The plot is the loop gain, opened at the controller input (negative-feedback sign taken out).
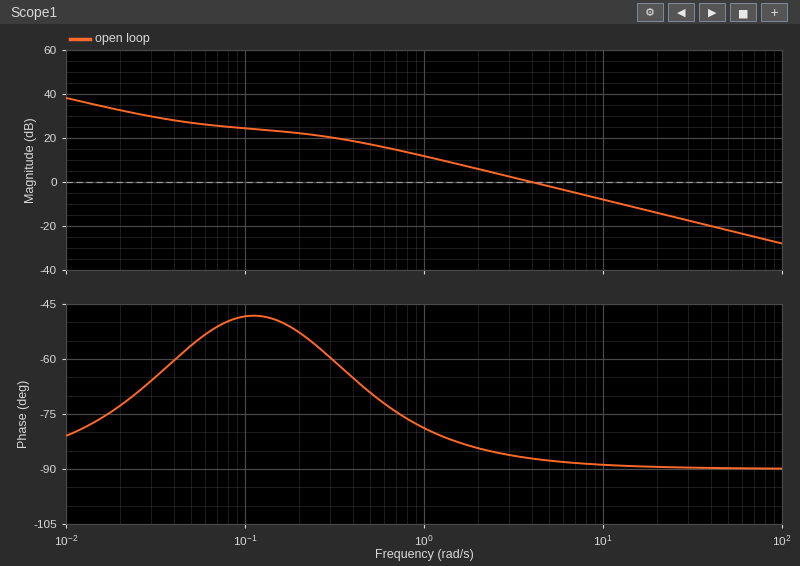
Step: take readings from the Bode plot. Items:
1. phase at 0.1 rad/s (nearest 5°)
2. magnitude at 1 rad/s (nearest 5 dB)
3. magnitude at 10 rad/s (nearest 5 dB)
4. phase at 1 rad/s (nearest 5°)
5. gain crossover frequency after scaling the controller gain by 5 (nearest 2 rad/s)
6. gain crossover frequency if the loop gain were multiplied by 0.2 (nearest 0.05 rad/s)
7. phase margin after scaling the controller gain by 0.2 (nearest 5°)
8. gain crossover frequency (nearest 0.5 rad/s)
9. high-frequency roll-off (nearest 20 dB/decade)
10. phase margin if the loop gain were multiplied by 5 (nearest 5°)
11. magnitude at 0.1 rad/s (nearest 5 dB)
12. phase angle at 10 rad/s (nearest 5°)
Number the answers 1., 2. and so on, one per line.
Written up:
1. -50°
2. 10 dB
3. -10 dB
4. -80°
5. 20 rad/s
6. 0.75 rad/s
7. 105°
8. 4.0 rad/s
9. -20 dB/decade
10. 90°
11. 25 dB
12. -90°
